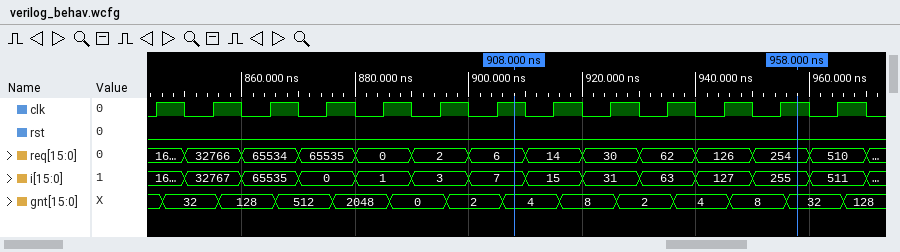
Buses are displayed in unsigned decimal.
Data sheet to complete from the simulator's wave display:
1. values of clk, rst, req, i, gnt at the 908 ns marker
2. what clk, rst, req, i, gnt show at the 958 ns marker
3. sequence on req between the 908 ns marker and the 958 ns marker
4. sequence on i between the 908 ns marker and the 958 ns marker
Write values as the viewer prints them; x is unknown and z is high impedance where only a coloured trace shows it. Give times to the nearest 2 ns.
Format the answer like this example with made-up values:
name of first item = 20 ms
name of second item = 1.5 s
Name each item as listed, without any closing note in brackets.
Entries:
values of clk, rst, req, i, gnt at the 908 ns marker = clk=1, rst=0, req=6, i=7, gnt=4
what clk, rst, req, i, gnt show at the 958 ns marker = clk=1, rst=0, req=254, i=255, gnt=32
sequence on req between the 908 ns marker and the 958 ns marker = 6, 14, 30, 62, 126, 254
sequence on i between the 908 ns marker and the 958 ns marker = 7, 15, 31, 63, 127, 255
